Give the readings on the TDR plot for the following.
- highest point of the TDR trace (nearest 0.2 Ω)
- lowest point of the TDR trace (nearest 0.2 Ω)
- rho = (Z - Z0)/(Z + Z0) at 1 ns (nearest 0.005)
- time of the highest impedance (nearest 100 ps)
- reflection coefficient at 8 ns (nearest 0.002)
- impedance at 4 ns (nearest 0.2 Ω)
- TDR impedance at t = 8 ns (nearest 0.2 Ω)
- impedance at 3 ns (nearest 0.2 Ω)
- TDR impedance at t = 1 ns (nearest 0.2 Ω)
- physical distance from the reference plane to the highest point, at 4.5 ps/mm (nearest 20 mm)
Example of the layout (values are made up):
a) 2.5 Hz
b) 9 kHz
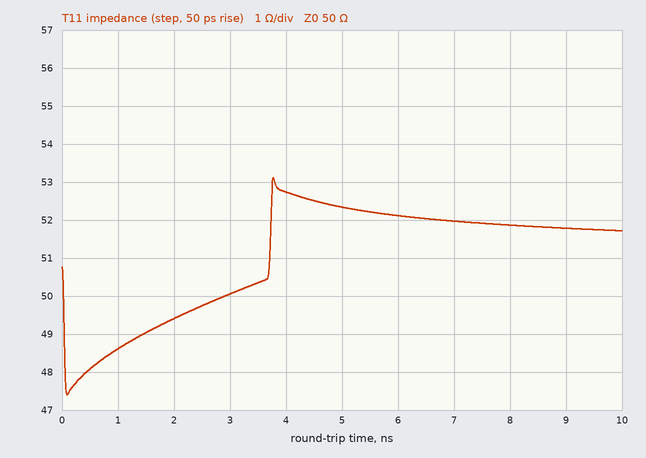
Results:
a) 53.2 Ω
b) 47.4 Ω
c) -0.015
d) 3.8 ns
e) +0.018
f) 52.8 Ω
g) 51.8 Ω
h) 50.0 Ω
i) 48.6 Ω
j) 420 mm
